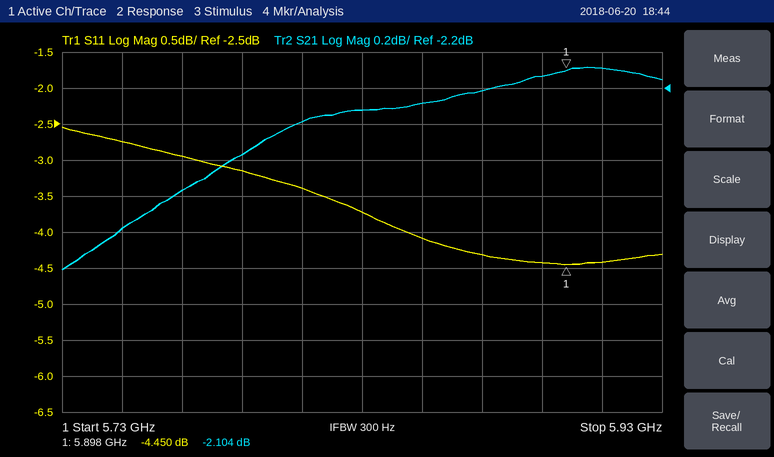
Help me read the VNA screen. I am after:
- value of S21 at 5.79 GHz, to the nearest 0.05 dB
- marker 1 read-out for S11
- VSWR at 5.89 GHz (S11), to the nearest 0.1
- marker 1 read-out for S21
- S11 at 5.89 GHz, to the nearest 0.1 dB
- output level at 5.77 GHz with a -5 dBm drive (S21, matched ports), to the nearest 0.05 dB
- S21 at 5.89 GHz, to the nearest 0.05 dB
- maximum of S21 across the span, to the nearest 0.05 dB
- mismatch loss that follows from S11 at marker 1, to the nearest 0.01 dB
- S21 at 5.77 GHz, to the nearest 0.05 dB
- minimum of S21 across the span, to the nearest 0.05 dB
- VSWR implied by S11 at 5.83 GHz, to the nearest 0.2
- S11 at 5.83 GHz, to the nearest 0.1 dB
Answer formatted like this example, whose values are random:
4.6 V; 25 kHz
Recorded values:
-2.55 dB; -4.450 dB; 4.0; -2.104 dB; -4.4 dB; -7.75 dBm; -2.15 dB; -2.10 dB; 1.93 dB; -2.75 dB; -3.20 dB; 4.8; -3.7 dB
